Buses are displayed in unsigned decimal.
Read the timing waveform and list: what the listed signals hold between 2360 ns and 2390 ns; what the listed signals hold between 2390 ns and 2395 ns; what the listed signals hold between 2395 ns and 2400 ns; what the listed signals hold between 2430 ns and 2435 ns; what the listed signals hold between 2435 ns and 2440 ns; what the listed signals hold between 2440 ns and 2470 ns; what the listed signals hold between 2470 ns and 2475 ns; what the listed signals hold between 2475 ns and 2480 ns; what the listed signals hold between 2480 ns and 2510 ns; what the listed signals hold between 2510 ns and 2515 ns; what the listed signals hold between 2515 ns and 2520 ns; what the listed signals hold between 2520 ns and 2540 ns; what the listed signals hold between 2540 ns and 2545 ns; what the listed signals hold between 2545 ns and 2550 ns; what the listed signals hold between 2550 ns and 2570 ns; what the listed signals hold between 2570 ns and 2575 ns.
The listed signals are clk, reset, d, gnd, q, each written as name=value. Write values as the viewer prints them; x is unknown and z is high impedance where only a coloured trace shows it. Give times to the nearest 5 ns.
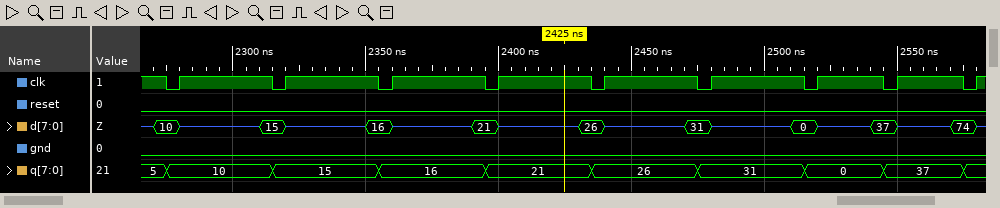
clk=1, reset=0, d=z, gnd=0, q=16
clk=1, reset=0, d=21, gnd=0, q=16
clk=0, reset=0, d=21, gnd=0, q=21
clk=1, reset=0, d=26, gnd=0, q=21
clk=0, reset=0, d=26, gnd=0, q=26
clk=1, reset=0, d=z, gnd=0, q=26
clk=1, reset=0, d=31, gnd=0, q=26
clk=0, reset=0, d=31, gnd=0, q=31
clk=1, reset=0, d=z, gnd=0, q=31
clk=1, reset=0, d=0, gnd=0, q=31
clk=0, reset=0, d=0, gnd=0, q=0
clk=1, reset=0, d=z, gnd=0, q=0
clk=1, reset=0, d=37, gnd=0, q=0
clk=0, reset=0, d=37, gnd=0, q=37
clk=1, reset=0, d=z, gnd=0, q=37
clk=1, reset=0, d=74, gnd=0, q=37
